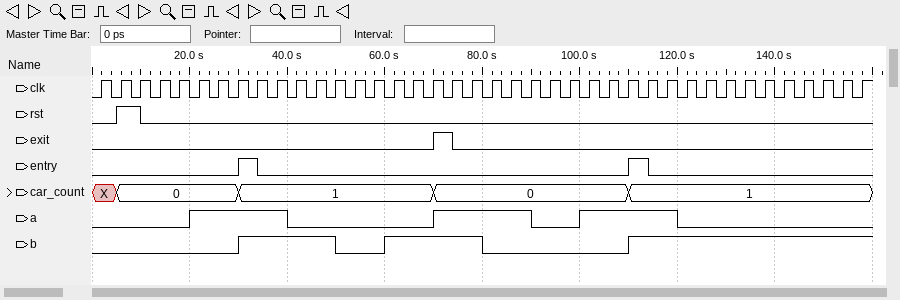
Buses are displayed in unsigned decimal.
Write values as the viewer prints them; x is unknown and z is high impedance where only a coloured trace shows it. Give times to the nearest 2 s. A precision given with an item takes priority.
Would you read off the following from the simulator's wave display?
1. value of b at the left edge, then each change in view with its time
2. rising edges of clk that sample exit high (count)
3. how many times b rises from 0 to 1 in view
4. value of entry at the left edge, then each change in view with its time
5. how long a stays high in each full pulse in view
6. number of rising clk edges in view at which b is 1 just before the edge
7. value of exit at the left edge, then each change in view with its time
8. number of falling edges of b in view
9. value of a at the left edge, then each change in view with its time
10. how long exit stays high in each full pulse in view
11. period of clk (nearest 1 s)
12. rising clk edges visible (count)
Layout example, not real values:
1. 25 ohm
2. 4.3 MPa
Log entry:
1. 0, 1 at 30 s, 0 at 50 s, 1 at 60 s, 0 at 80 s, 1 at 110 s
2. 1
3. 3
4. 0, 1 at 30 s, 0 at 34 s, 1 at 110 s, 0 at 114 s
5. 20 s, 20 s, 20 s
6. 22
7. 0, 1 at 70 s, 0 at 74 s
8. 2
9. 0, 1 at 20 s, 0 at 40 s, 1 at 70 s, 0 at 90 s, 1 at 100 s, 0 at 120 s
10. 4 s
11. 4 s
12. 40
